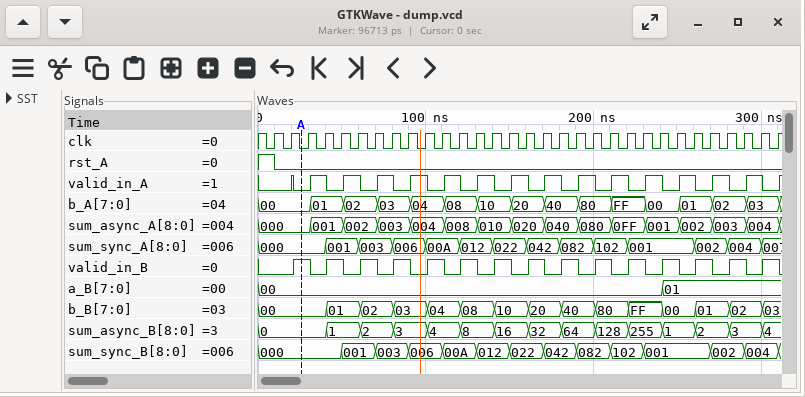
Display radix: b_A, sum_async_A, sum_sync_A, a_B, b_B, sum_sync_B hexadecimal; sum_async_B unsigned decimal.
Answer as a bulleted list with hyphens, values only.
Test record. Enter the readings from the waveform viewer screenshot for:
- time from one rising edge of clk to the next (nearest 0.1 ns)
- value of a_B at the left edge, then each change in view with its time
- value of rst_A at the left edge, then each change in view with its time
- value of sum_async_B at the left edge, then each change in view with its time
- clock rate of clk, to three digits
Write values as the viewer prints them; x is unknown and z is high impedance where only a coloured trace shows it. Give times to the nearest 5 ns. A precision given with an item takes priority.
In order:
- 10 ns
- 00, 01 at 240 ns
- 1, 0 at 10 ns
- 0, 1 at 40 ns, 2 at 60 ns, 3 at 80 ns, 4 at 100 ns, 8 at 120 ns, 16 at 140 ns, 32 at 160 ns, 64 at 180 ns, 128 at 200 ns, 255 at 220 ns, 1 at 240 ns, 2 at 260 ns, 3 at 280 ns, 4 at 300 ns
- 100 MHz
